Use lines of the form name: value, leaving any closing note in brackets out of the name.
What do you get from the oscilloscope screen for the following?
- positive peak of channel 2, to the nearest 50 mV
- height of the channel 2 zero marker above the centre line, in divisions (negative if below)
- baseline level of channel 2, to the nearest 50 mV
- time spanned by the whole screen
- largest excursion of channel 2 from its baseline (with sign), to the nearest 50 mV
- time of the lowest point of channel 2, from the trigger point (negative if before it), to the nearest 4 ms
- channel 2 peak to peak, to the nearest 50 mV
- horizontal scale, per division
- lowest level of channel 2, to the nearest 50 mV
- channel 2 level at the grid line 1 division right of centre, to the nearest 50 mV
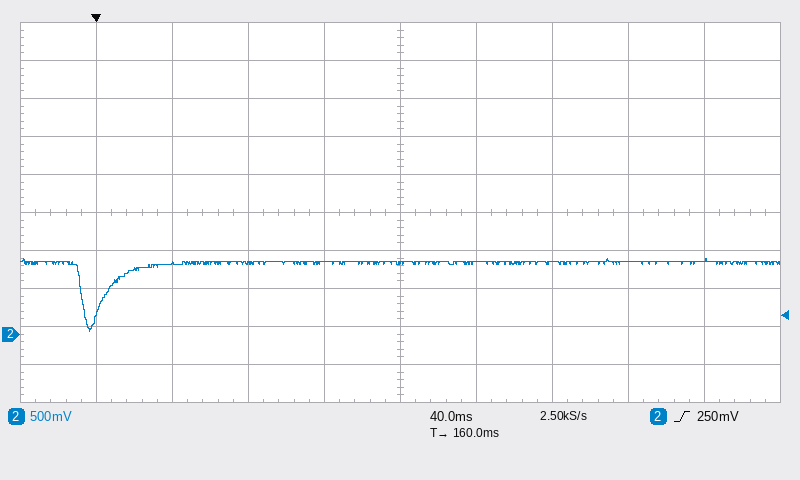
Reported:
positive peak of channel 2, to the nearest 50 mV: 1.00 V
height of the channel 2 zero marker above the centre line, in divisions: -3.2 div
baseline level of channel 2, to the nearest 50 mV: 950 mV
time spanned by the whole screen: 400 ms
largest excursion of channel 2 from its baseline (with sign), to the nearest 50 mV: -900 mV
time of the lowest point of channel 2, from the trigger point (negative if before it), to the nearest 4 ms: -4 ms
channel 2 peak to peak, to the nearest 50 mV: 950 mV
horizontal scale, per division: 40 ms
lowest level of channel 2, to the nearest 50 mV: 50 mV
channel 2 level at the grid line 1 division right of centre, to the nearest 50 mV: 950 mV
